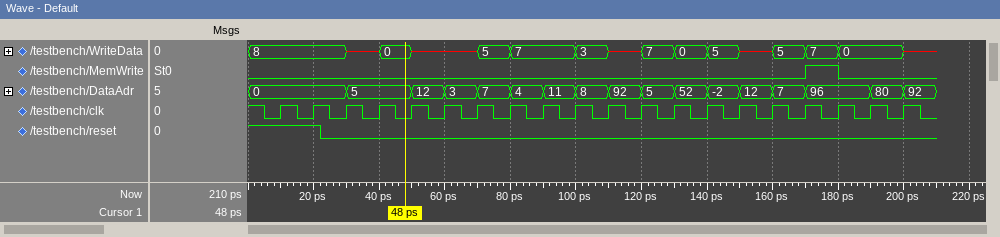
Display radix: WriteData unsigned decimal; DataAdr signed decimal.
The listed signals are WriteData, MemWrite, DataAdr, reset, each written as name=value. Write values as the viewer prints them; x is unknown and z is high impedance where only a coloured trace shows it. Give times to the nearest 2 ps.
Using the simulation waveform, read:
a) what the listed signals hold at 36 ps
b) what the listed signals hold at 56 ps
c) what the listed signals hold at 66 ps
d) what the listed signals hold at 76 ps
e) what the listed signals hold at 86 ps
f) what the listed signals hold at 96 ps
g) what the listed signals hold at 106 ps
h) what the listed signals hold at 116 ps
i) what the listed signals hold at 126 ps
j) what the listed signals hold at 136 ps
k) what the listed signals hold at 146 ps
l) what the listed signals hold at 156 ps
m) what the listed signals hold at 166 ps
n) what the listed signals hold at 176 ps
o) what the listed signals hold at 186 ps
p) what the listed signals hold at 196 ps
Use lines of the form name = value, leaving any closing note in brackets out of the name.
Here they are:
what the listed signals hold at 36 ps = WriteData=x, MemWrite=0, DataAdr=5, reset=0
what the listed signals hold at 56 ps = WriteData=x, MemWrite=0, DataAdr=12, reset=0
what the listed signals hold at 66 ps = WriteData=x, MemWrite=0, DataAdr=3, reset=0
what the listed signals hold at 76 ps = WriteData=5, MemWrite=0, DataAdr=7, reset=0
what the listed signals hold at 86 ps = WriteData=7, MemWrite=0, DataAdr=4, reset=0
what the listed signals hold at 96 ps = WriteData=7, MemWrite=0, DataAdr=11, reset=0
what the listed signals hold at 106 ps = WriteData=3, MemWrite=0, DataAdr=8, reset=0
what the listed signals hold at 116 ps = WriteData=x, MemWrite=0, DataAdr=92, reset=0
what the listed signals hold at 126 ps = WriteData=7, MemWrite=0, DataAdr=5, reset=0
what the listed signals hold at 136 ps = WriteData=0, MemWrite=0, DataAdr=52, reset=0
what the listed signals hold at 146 ps = WriteData=5, MemWrite=0, DataAdr=-2, reset=0
what the listed signals hold at 156 ps = WriteData=x, MemWrite=0, DataAdr=12, reset=0
what the listed signals hold at 166 ps = WriteData=5, MemWrite=0, DataAdr=7, reset=0
what the listed signals hold at 176 ps = WriteData=7, MemWrite=1, DataAdr=96, reset=0
what the listed signals hold at 186 ps = WriteData=0, MemWrite=0, DataAdr=96, reset=0
what the listed signals hold at 196 ps = WriteData=0, MemWrite=0, DataAdr=80, reset=0
